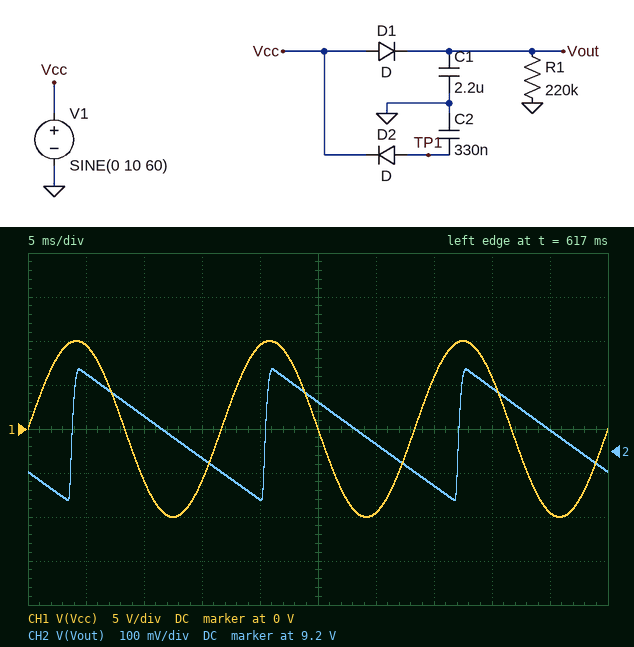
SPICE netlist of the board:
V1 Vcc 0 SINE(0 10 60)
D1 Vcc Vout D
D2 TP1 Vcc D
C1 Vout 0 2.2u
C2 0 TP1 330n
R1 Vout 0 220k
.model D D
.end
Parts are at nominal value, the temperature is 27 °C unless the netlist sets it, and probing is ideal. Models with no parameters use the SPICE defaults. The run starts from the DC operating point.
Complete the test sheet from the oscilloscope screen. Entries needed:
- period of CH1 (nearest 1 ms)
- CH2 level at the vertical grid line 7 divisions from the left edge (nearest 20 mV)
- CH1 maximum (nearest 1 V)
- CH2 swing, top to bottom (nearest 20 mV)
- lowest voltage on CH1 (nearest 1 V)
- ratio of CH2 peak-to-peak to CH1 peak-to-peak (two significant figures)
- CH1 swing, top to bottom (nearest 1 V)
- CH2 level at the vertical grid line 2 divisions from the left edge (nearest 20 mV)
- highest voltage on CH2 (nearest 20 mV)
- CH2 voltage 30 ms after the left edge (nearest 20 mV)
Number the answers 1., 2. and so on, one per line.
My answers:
1. 17 ms
2. 9.12 V
3. 10 V
4. 300 mV
5. -10 V
6. 0.015
7. 20 V
8. 9.28 V
9. 9.38 V
10. 9.22 V
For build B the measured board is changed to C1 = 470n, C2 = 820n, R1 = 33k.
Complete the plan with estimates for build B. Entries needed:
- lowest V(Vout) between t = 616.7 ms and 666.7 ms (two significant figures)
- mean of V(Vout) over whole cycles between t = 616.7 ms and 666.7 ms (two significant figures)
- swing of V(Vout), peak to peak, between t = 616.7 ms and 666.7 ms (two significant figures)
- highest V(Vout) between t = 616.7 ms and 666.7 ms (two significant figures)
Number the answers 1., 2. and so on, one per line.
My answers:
1. 3.9 V
2. 6.5 V
3. 5.4 V
4. 9.4 V
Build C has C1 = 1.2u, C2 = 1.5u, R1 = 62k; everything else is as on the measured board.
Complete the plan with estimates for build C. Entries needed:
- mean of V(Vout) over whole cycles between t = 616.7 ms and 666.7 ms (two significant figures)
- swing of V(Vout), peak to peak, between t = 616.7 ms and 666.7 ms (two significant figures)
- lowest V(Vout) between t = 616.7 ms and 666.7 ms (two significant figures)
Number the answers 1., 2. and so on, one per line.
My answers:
1. 8.5 V
2. 1.7 V
3. 7.7 V
